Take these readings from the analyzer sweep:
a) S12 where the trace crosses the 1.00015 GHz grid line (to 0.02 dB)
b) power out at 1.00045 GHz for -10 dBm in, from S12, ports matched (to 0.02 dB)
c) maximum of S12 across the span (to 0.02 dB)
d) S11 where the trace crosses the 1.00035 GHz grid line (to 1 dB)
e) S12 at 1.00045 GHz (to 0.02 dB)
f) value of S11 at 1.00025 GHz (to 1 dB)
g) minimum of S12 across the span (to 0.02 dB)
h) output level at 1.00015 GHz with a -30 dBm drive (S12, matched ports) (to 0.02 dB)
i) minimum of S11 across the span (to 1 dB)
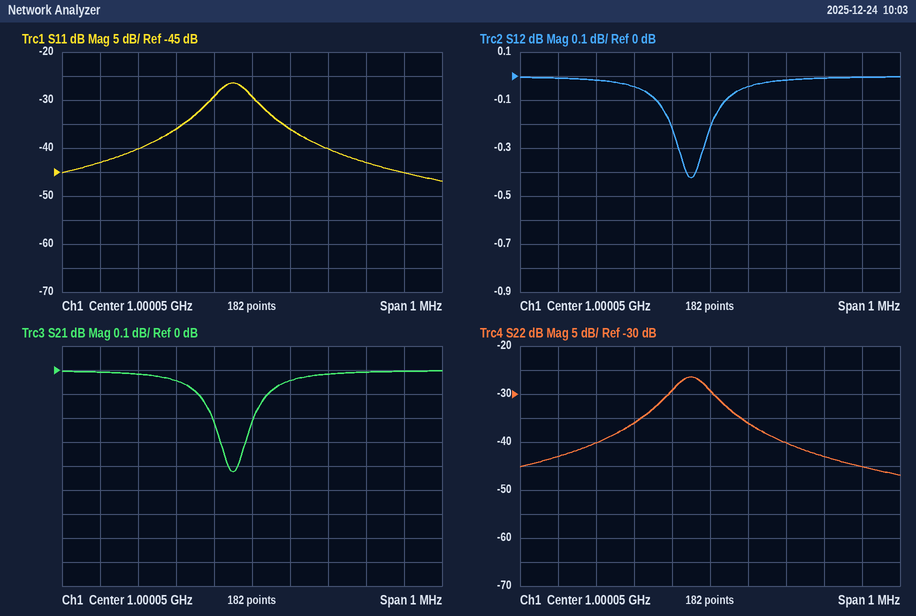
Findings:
-0.04 dB
-10.00 dBm
0.00 dB
-43 dB
0.00 dB
-40 dB
-0.42 dB
-30.04 dBm
-47 dB
